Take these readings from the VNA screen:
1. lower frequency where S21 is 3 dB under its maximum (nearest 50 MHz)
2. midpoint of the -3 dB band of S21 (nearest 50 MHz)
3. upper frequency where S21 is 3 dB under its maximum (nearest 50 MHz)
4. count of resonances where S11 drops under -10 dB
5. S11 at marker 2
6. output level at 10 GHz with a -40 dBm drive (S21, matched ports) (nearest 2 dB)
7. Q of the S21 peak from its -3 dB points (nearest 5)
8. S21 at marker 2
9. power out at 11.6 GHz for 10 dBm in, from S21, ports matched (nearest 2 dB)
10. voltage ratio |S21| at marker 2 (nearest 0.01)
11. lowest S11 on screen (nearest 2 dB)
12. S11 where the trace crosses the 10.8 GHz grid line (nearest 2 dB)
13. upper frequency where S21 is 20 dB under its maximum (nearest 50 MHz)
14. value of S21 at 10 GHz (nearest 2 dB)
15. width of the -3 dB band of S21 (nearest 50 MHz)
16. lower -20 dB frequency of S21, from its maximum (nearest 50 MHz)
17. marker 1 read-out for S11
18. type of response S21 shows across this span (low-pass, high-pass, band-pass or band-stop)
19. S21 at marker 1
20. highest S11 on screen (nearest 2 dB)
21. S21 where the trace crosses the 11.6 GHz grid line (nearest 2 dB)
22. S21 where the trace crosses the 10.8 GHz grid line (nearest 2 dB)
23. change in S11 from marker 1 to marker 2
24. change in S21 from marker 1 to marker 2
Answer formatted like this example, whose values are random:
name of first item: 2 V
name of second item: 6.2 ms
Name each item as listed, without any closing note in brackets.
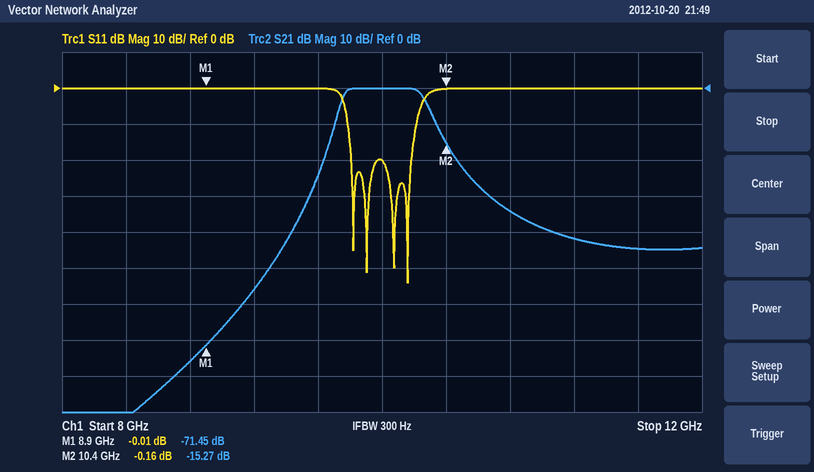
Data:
lower frequency where S21 is 3 dB under its maximum: 9.75 GHz
midpoint of the -3 dB band of S21: 10.00 GHz
upper frequency where S21 is 3 dB under its maximum: 10.25 GHz
count of resonances where S11 drops under -10 dB: 4
S11 at marker 2: -0.16 dB
output level at 10 GHz with a -40 dBm drive (S21, matched ports): -40 dBm
Q of the S21 peak from its -3 dB points: 20
S21 at marker 2: -15.27 dB
power out at 11.6 GHz for 10 dBm in, from S21, ports matched: -34 dBm
voltage ratio |S21| at marker 2: 0.17
lowest S11 on screen: -54 dB
S11 where the trace crosses the 10.8 GHz grid line: 0 dB
upper frequency where S21 is 20 dB under its maximum: 10.45 GHz
value of S21 at 10 GHz: 0 dB
width of the -3 dB band of S21: 500 MHz
lower -20 dB frequency of S21, from its maximum: 9.65 GHz
marker 1 read-out for S11: -0.01 dB
type of response S21 shows across this span: band-pass
S21 at marker 1: -71.45 dB
highest S11 on screen: 0 dB
S21 where the trace crosses the 11.6 GHz grid line: -44 dB
S21 where the trace crosses the 10.8 GHz grid line: -34 dB
change in S11 from marker 1 to marker 2: -0.15 dB
change in S21 from marker 1 to marker 2: 56.18 dB
